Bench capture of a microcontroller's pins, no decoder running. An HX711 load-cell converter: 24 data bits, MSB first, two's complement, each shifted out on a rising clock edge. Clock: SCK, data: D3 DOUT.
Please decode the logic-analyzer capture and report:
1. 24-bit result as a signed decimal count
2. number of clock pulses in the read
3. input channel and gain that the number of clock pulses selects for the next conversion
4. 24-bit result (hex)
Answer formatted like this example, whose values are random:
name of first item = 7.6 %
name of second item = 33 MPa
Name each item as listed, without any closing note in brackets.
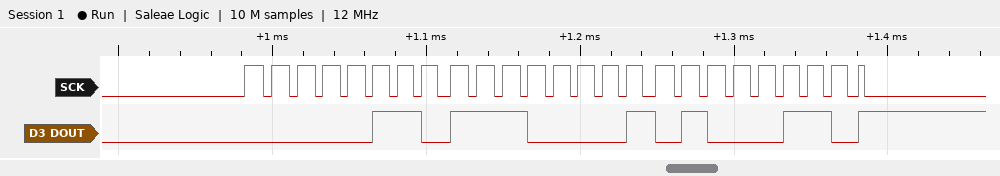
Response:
24-bit result as a signed decimal count = 450886
number of clock pulses in the read = 25
input channel and gain that the number of clock pulses selects for the next conversion = channel A, gain 128
24-bit result = 0x06E146
